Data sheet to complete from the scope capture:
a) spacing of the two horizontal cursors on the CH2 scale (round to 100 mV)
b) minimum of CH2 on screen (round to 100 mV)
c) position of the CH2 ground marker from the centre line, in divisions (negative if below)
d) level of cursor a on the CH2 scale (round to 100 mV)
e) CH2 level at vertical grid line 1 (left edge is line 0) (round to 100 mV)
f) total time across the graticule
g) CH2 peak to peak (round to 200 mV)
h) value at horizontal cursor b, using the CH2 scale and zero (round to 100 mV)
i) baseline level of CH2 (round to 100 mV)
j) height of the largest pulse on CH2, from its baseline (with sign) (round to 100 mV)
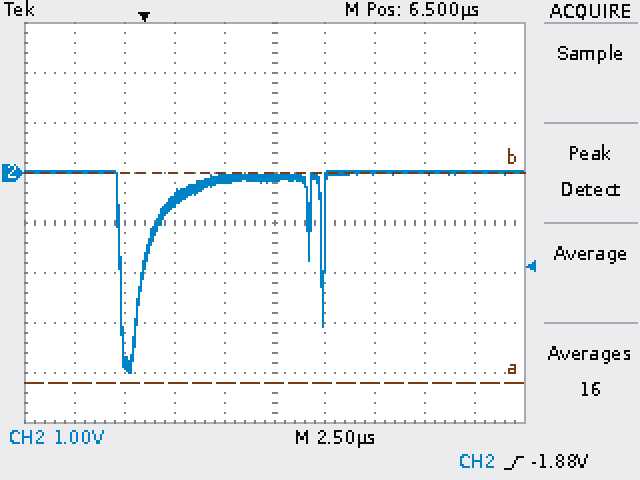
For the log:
4.2 V
-4.0 V
+1.0 div
-4.2 V
0.0 V
25 µs
4.0 V
0.0 V
0.0 V
-4.0 V
